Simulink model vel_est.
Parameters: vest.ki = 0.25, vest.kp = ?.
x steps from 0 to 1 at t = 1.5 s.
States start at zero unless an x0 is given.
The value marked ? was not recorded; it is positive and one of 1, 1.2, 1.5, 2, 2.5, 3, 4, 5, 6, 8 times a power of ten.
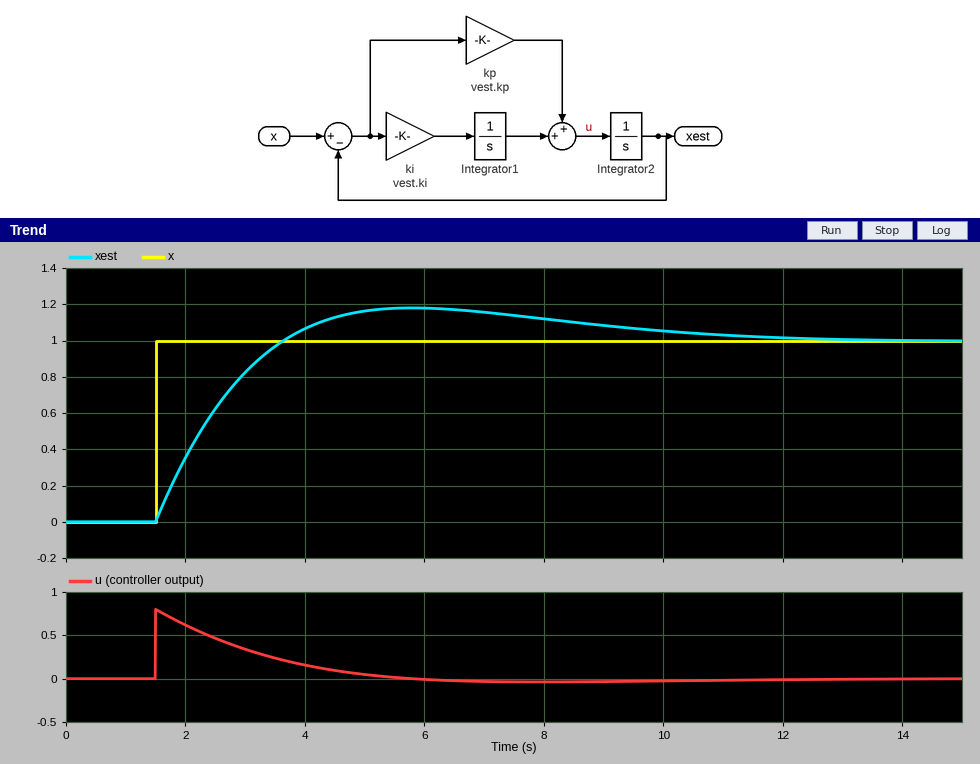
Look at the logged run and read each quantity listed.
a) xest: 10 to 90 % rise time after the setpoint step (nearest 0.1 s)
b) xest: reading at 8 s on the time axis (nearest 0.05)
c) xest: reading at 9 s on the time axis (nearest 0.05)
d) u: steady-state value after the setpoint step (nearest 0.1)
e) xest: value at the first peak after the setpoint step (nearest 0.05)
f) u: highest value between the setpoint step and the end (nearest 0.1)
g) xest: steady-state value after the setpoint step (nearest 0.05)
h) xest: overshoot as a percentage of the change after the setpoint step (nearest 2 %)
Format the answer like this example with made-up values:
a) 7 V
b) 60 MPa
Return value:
a) 1.6 s
b) 1.10
c) 1.10
d) 0.0
e) 1.20
f) 0.8
g) 1.00
h) 18 %
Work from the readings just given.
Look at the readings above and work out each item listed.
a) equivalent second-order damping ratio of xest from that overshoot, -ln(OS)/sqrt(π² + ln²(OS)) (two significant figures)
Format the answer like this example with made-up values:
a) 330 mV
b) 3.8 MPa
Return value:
a) 0.48
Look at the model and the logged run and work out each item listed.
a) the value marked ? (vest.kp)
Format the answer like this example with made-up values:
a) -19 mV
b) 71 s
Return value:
a) 0.8
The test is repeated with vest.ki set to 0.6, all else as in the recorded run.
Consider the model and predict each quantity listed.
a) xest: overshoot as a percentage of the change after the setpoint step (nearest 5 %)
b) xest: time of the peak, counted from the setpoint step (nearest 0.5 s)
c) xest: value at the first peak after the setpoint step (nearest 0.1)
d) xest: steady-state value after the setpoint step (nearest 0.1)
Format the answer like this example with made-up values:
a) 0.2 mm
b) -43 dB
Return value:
a) 30 %
b) 3.0 s
c) 1.3
d) 1.0
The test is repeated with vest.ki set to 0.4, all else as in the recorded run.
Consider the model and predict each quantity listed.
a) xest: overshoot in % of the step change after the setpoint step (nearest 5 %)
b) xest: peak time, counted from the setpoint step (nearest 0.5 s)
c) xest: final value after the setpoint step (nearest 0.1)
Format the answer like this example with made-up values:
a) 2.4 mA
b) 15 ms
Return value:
a) 25 %
b) 3.5 s
c) 1.0
